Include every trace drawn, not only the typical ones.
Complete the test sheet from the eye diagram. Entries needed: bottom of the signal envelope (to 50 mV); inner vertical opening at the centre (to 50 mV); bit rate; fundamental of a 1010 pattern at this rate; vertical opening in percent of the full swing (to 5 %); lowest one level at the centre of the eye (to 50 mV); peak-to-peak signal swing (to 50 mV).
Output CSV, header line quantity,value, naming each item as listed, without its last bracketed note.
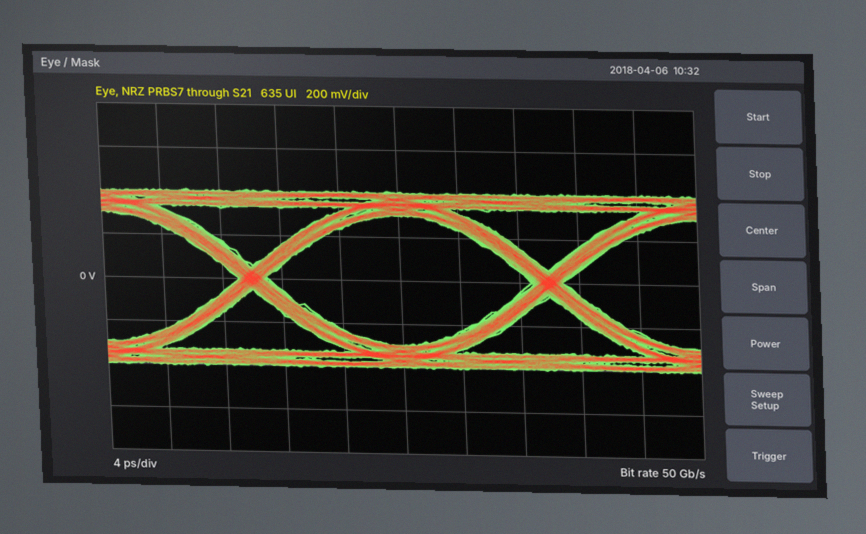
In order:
quantity,value
bottom of the signal envelope,-400 mV
inner vertical opening at the centre,600 mV
bit rate,50 Gb/s
fundamental of a 1010 pattern at this rate,25 GHz
vertical opening in percent of the full swing,75 %
lowest one level at the centre of the eye,300 mV
peak-to-peak signal swing,800 mV
